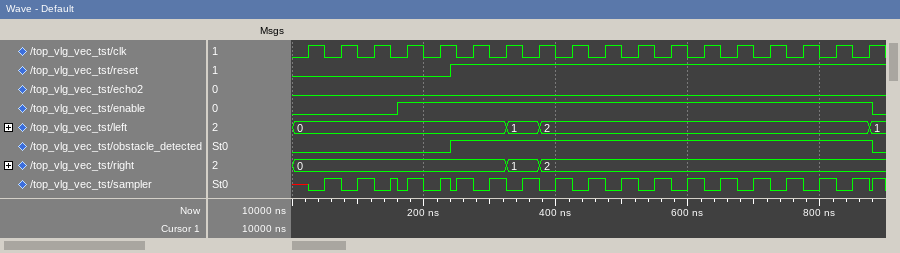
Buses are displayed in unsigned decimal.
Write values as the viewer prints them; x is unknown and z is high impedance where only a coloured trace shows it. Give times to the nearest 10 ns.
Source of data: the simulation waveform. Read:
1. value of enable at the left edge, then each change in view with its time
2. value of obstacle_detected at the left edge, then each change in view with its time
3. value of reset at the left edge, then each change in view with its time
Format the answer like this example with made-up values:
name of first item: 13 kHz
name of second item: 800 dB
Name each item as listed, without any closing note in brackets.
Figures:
value of enable at the left edge, then each change in view with its time: 0, 1 at 160 ns, 0 at 880 ns
value of obstacle_detected at the left edge, then each change in view with its time: 0, 1 at 240 ns, 0 at 880 ns
value of reset at the left edge, then each change in view with its time: 0, 1 at 240 ns
